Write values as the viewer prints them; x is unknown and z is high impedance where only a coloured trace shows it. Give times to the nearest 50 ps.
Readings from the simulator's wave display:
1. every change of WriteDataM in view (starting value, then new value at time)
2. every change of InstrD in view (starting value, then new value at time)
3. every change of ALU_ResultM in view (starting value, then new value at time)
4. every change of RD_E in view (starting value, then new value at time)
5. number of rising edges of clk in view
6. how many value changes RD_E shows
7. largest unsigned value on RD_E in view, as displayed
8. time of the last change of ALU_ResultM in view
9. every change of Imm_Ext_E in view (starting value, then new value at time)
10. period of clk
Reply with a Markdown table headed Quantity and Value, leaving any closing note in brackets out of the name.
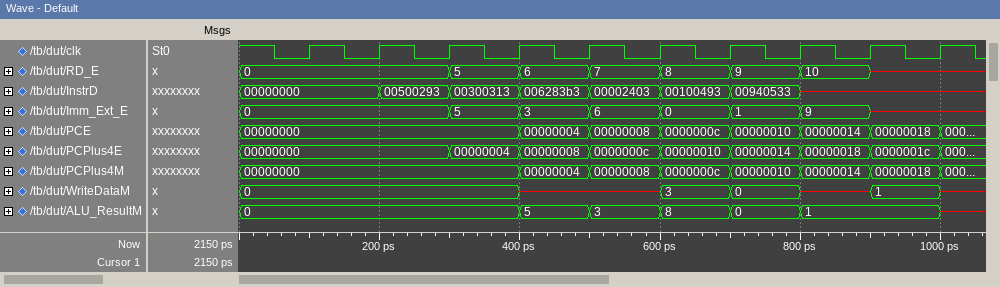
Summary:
| Quantity | Value |
|---|---|
| every change of WriteDataM in view | 0, x at 400 ps, 3 at 600 ps, 0 at 700 ps, x at 800 ps, 1 at 900 ps, x at 1000 ps |
| every change of InstrD in view | 00000000, 00500293 at 200 ps, 00300313 at 300 ps, 006283b3 at 400 ps, 00002403 at 500 ps, 00100493 at 600 ps, 00940533 at 700 ps, x at 800 ps |
| every change of ALU_ResultM in view | 0, 5 at 400 ps, 3 at 500 ps, 8 at 600 ps, 0 at 700 ps, 1 at 800 ps, x at 1000 ps |
| every change of RD_E in view | 0, 5 at 300 ps, 6 at 400 ps, 7 at 500 ps, 8 at 600 ps, 9 at 700 ps, 10 at 800 ps, x at 900 ps |
| number of rising edges of clk in view | 10 |
| how many value changes RD_E shows | 7 |
| largest unsigned value on RD_E in view, as displayed | 10 |
| time of the last change of ALU_ResultM in view | 1000 ps |
| every change of Imm_Ext_E in view | 0, 5 at 300 ps, 3 at 400 ps, 6 at 500 ps, 0 at 600 ps, 1 at 700 ps, 9 at 800 ps, x at 900 ps |
| period of clk | 100 ps |
